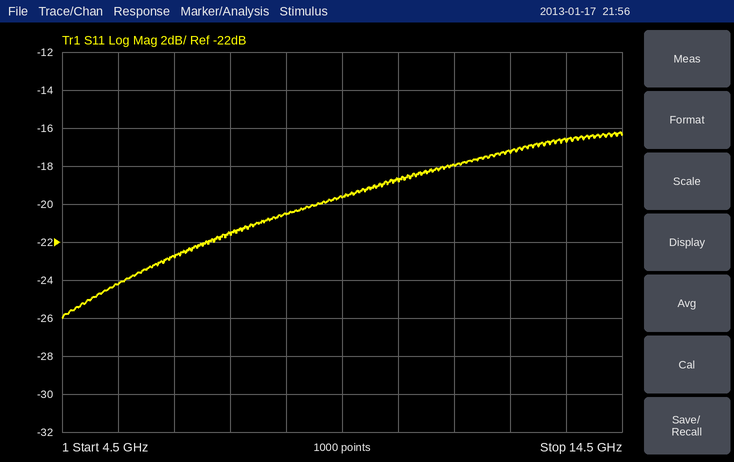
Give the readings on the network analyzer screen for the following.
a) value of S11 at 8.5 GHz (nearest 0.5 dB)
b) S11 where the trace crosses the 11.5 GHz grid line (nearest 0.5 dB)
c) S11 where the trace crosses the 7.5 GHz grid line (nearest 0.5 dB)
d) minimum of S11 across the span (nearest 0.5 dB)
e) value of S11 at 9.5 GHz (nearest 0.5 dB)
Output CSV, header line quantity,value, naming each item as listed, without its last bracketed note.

quantity,value
value of S11 at 8.5 GHz,-20.5 dB
S11 where the trace crosses the 11.5 GHz grid line,-18.0 dB
S11 where the trace crosses the 7.5 GHz grid line,-21.5 dB
minimum of S11 across the span,-26.0 dB
value of S11 at 9.5 GHz,-19.5 dB
